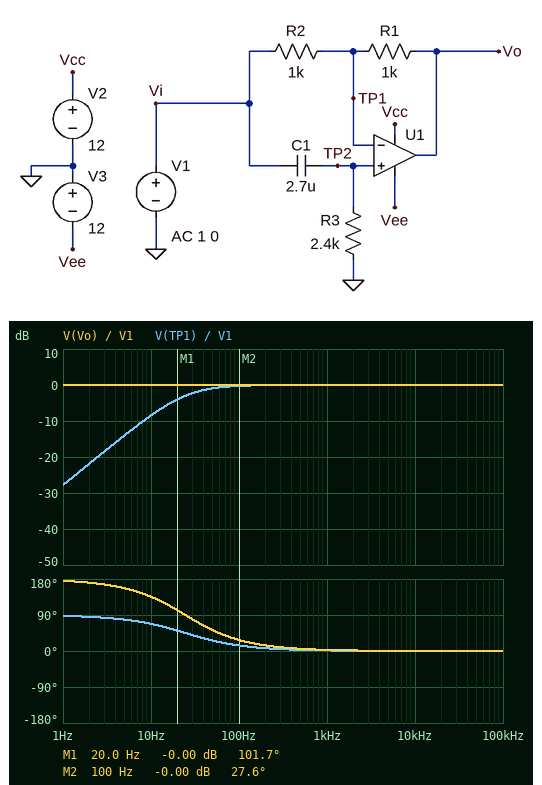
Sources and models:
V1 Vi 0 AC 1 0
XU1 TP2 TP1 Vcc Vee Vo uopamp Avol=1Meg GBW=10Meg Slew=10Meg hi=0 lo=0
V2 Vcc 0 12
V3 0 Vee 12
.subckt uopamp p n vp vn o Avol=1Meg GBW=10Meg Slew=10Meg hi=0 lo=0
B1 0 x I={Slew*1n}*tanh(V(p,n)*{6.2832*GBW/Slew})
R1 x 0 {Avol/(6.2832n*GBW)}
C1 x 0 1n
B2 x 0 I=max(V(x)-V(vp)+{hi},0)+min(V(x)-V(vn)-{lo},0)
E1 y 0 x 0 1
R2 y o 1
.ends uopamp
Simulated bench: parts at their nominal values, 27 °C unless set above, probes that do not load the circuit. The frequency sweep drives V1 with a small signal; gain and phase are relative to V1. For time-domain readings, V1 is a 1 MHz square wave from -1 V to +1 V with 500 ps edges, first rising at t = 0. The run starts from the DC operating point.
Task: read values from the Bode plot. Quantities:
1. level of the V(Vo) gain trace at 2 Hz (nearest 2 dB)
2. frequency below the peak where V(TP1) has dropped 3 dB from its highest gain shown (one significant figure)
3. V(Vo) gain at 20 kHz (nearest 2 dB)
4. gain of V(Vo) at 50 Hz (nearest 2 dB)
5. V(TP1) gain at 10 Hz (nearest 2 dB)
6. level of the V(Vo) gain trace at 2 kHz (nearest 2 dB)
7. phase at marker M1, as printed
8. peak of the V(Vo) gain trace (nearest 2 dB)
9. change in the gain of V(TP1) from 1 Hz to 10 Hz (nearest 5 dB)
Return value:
0 dB
20 Hz
0 dB
0 dB
-8 dB
0 dB
101.7 deg
0 dB
20 dB
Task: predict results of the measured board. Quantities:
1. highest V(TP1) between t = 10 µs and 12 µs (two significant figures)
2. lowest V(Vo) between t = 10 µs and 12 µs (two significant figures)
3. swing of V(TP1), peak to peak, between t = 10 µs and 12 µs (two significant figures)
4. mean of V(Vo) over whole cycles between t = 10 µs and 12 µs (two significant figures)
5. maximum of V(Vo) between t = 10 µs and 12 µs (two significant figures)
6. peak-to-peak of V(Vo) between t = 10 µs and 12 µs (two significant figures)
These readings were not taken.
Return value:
2.0 V
1.0 V
2.0 V
2.0 V
3.0 V
2.0 V
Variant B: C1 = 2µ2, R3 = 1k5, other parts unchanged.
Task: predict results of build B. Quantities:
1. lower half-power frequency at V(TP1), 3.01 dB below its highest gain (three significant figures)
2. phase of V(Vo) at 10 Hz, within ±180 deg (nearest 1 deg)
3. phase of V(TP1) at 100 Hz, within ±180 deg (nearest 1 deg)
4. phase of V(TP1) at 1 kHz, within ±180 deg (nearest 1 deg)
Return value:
48.2 Hz
157 deg
26 deg
3 deg
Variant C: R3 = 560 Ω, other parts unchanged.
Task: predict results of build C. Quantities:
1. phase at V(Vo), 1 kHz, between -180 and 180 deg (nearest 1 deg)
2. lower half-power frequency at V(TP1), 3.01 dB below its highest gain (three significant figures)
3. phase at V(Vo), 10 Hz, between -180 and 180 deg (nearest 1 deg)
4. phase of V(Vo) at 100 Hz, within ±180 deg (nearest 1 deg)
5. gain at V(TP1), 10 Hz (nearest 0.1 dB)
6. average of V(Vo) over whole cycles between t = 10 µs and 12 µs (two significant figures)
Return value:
12 deg
105 Hz
169 deg
93 deg
-20.5 dB
2.0 V
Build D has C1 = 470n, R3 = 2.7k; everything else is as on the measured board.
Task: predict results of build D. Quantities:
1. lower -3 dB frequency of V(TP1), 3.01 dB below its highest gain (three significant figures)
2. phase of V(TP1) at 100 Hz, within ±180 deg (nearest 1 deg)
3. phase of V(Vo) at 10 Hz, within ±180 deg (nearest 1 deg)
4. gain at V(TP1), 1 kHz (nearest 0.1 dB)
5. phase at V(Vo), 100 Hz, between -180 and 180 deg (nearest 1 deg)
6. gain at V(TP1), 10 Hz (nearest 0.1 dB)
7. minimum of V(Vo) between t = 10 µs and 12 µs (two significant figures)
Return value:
125 Hz
51 deg
171 deg
-0.1 dB
103 deg
-22.0 dB
980 mV
